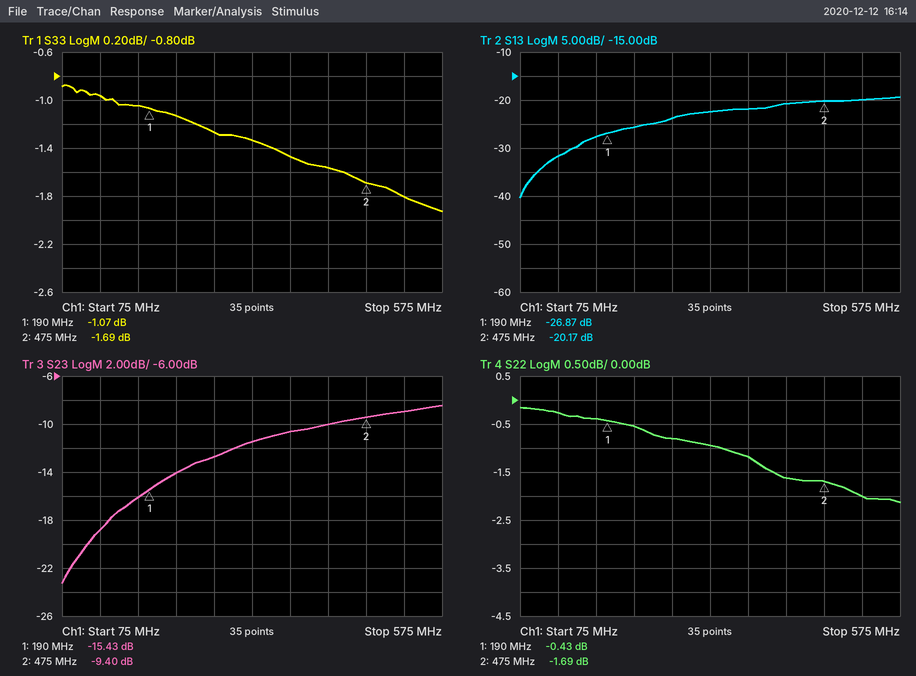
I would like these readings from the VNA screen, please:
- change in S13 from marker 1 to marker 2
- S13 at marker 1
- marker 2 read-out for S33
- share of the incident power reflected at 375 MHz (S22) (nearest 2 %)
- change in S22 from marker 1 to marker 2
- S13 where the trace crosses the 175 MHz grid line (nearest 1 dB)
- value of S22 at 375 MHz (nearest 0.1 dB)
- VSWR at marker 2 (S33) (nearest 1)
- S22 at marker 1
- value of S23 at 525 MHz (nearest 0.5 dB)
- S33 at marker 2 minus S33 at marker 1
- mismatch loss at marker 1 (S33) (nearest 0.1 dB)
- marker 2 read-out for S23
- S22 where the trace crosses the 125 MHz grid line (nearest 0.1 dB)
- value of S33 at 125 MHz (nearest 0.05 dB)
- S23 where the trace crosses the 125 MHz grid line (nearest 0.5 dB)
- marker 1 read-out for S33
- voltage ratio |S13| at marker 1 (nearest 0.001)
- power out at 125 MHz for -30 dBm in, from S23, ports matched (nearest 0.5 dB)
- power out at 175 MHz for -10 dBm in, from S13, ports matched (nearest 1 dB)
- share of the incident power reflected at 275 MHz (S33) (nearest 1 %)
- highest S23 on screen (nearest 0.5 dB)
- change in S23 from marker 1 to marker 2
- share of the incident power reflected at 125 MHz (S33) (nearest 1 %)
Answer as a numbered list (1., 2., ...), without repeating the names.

1. 6.70 dB
2. -26.87 dB
3. -1.69 dB
4. 76 %
5. -1.26 dB
6. -28 dB
7. -1.2 dB
8. 10
9. -0.43 dB
10. -9.0 dB
11. -0.62 dB
12. 6.6 dB
13. -9.40 dB
14. -0.3 dB
15. -0.95 dB
16. -19.0 dB
17. -1.07 dB
18. 0.045
19. -49.0 dBm
20. -38 dBm
21. 75 %
22. -8.5 dB
23. 6.03 dB
24. 80 %
